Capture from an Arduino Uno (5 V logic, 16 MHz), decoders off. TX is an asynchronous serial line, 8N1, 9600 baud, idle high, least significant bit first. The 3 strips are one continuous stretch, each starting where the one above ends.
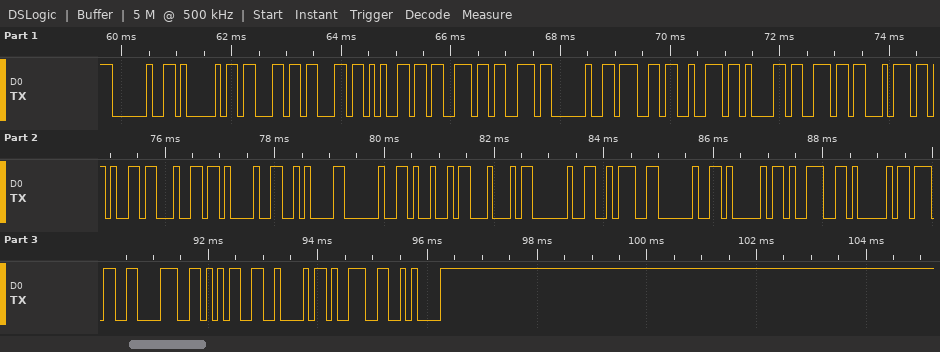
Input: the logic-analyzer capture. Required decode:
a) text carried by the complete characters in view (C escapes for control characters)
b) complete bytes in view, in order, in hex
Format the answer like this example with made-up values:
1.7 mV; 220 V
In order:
" Access granted!\n ID : A9A785B9\n"; 20 41 63 63 65 73 73 20 67 72 61 6E 74 65 64 21 0A 20 49 44 20 3A 20 41 39 41 37 38 35 42 39 0A
